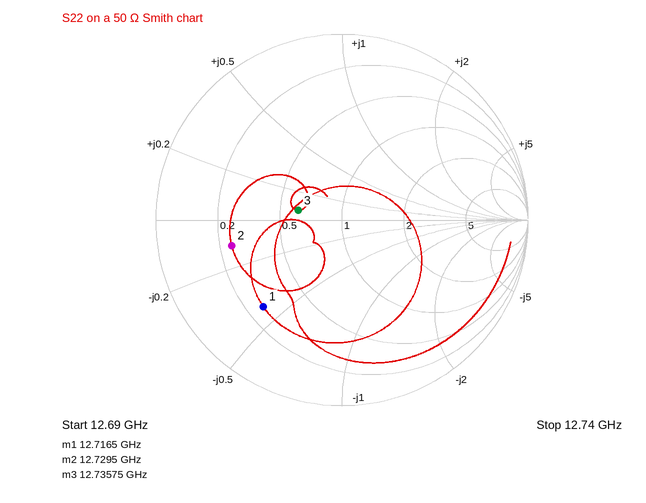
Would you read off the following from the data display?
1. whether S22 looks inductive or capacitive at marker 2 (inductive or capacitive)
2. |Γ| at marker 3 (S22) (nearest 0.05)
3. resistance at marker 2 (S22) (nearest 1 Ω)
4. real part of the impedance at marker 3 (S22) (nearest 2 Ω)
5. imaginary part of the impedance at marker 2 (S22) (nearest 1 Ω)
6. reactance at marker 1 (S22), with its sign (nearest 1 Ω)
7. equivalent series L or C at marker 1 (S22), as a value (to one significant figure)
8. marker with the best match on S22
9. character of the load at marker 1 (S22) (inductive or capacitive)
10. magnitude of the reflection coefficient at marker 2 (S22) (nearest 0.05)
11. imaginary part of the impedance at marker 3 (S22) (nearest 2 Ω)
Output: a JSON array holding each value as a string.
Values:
["capacitive", "0.25", "12 Ω", "30 Ω", "-5 Ω", "-21 Ω", "600 fF", "marker 3", "capacitive", "0.60", "+4 Ω"]
